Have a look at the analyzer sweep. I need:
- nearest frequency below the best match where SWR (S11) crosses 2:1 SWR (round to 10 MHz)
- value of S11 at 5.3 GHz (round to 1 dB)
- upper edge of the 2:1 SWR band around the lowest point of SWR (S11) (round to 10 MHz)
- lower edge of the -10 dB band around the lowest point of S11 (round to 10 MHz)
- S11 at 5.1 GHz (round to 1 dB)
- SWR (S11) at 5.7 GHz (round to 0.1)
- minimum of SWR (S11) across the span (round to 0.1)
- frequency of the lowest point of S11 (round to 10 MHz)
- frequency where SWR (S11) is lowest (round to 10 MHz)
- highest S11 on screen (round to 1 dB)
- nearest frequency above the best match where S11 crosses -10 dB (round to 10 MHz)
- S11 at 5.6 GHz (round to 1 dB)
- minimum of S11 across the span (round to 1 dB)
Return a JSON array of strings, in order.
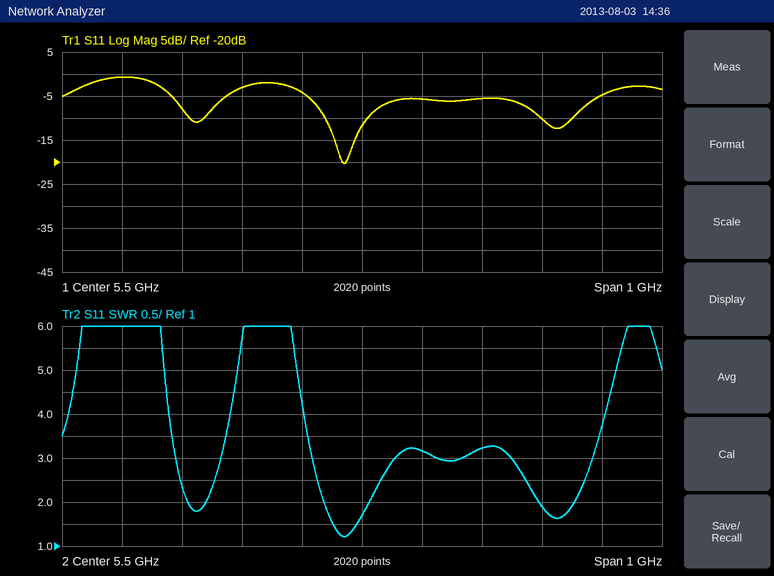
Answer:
["5.44 GHz", "-3 dB", "5.51 GHz", "5.44 GHz", "-1 dB", "3.2", "1.2", "5.47 GHz", "5.47 GHz", "-1 dB", "5.51 GHz", "-6 dB", "-20 dB"]
